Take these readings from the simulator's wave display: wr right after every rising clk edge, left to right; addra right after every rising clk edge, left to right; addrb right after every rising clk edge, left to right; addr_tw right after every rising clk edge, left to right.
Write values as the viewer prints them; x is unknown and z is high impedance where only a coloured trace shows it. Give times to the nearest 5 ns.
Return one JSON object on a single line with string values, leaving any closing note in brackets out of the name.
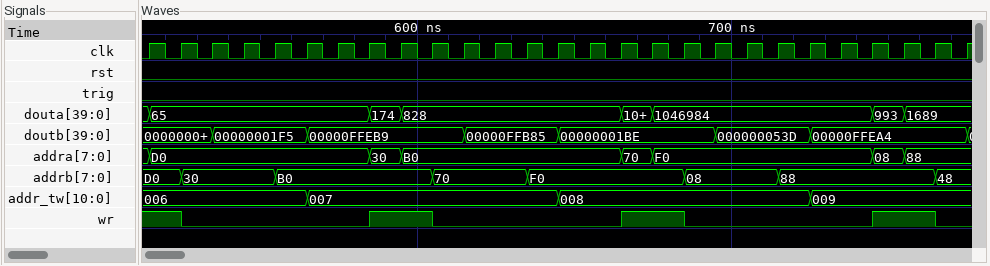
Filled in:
{"wr right after every rising clk edge, left to right": "1 0 0 0 0 0 0 1 1 0 0 0 0 0 0 1 1 0 0 0 0 0 0 1 1 0 0", "addra right after every rising clk edge, left to right": "D0, D0, D0, D0, D0, D0, D0, 30, B0, B0, B0, B0, B0, B0, B0, 70, F0, F0, F0, F0, F0, F0, F0, 08, 88, 88, 88", "addrb right after every rising clk edge, left to right": "D0, 30, 30, 30, B0, B0, B0, B0, B0, 70, 70, 70, F0, F0, F0, F0, F0, 08, 08, 08, 88, 88, 88, 88, 88, 48, 48", "addr_tw right after every rising clk edge, left to right": "006, 006, 006, 006, 006, 007, 007, 007, 007, 007, 007, 007, 007, 008, 008, 008, 008, 008, 008, 008, 008, 009, 009, 009, 009, 009, 009"}
